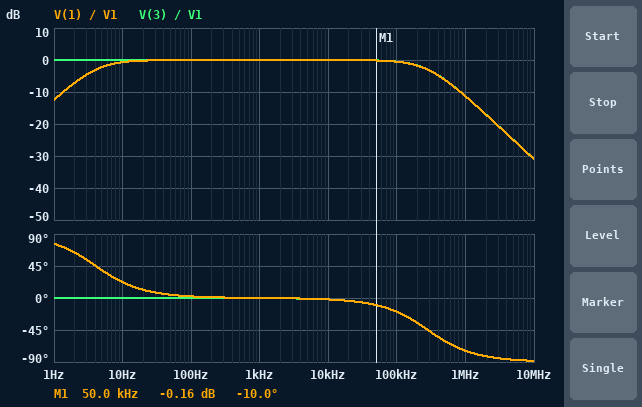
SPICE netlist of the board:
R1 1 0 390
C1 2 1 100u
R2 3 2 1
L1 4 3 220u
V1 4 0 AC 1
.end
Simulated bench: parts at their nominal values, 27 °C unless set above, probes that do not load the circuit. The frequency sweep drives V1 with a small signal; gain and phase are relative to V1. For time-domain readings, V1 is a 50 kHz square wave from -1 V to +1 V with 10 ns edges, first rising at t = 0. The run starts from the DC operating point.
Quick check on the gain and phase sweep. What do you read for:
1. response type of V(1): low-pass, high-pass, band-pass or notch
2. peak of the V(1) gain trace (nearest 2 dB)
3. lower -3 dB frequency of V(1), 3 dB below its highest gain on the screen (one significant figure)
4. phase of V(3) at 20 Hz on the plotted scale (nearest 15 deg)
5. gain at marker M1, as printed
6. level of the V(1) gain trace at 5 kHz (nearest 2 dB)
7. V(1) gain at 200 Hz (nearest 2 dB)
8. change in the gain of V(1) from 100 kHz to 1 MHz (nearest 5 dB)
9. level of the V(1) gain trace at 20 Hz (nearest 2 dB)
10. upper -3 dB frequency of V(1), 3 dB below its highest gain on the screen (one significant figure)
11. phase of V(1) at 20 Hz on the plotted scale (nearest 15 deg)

band-pass
0 dB
4 Hz
0 deg
-0.16 dB
0 dB
0 dB
-10 dB
0 dB
300 kHz
15 deg
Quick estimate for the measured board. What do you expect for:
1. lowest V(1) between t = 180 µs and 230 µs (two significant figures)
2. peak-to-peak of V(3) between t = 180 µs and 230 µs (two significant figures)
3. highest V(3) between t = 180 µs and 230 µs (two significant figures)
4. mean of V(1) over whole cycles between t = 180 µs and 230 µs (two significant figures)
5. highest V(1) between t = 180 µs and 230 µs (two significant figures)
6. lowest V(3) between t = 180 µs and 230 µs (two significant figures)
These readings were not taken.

-5.6 mV
2.0 V
1.0 V
990 mV
2.0 V
-1.0 V
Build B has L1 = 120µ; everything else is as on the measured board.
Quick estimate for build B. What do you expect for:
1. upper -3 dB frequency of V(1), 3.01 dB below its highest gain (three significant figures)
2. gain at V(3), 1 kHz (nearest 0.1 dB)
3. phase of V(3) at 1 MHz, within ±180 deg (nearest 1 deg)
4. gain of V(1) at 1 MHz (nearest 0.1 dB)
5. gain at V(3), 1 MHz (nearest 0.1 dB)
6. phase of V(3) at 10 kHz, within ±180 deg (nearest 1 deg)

519 kHz
0 dB
-63 deg
-6.8 dB
-6.7 dB
-1 deg
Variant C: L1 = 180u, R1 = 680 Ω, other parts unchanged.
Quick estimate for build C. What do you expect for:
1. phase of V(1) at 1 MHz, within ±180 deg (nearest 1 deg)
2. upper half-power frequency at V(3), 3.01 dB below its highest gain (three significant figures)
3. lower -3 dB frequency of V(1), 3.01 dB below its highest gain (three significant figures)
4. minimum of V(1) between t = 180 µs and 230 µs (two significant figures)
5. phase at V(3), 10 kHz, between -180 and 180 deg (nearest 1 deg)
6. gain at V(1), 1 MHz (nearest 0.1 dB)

-59 deg
602 kHz
2.34 Hz
-3.2 mV
-1 deg
-5.8 dB
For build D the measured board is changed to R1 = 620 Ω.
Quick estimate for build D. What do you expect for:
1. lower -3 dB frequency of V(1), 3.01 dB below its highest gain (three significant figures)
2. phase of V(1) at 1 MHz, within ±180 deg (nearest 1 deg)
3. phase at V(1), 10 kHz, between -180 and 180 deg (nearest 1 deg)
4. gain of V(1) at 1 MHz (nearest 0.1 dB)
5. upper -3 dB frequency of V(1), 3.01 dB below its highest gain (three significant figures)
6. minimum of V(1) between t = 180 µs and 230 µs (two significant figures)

2.56 Hz
-66 deg
-1 deg
-7.8 dB
449 kHz
-3.5 mV
